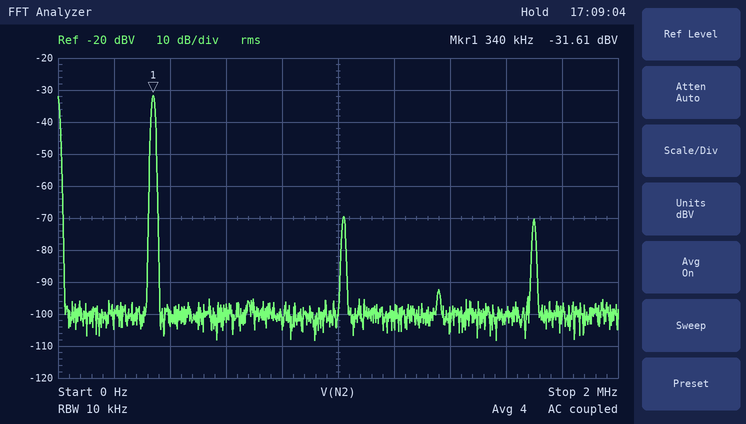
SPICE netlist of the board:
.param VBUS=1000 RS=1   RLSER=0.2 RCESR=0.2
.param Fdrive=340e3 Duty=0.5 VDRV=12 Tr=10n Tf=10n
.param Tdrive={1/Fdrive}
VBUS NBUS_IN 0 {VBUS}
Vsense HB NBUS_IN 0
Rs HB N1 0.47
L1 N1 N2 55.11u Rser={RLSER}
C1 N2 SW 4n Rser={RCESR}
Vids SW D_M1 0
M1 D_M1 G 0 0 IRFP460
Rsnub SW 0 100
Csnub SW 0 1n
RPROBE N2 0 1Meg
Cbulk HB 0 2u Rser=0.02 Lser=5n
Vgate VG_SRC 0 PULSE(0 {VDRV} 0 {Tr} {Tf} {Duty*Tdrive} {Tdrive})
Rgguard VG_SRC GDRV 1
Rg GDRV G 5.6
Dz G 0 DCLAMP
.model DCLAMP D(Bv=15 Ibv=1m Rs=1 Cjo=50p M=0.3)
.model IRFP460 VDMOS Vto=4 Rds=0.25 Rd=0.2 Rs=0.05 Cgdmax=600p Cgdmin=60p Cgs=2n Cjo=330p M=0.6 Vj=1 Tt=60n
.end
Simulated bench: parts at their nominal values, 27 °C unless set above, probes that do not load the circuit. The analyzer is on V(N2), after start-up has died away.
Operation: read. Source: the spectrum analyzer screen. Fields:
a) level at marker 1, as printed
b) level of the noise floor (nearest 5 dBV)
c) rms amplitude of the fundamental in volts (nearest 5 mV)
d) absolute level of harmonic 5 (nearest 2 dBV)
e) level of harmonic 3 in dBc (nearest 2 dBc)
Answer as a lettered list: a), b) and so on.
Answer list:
a) -31.61 dBV
b) -100 dBV
c) 25 mV
d) -70 dBV
e) -38 dBc
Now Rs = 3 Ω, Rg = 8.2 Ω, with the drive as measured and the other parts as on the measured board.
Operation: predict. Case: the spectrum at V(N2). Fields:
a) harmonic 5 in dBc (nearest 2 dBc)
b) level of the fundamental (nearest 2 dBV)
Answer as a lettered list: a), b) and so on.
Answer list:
a) -30 dBc
b) -42 dBV
